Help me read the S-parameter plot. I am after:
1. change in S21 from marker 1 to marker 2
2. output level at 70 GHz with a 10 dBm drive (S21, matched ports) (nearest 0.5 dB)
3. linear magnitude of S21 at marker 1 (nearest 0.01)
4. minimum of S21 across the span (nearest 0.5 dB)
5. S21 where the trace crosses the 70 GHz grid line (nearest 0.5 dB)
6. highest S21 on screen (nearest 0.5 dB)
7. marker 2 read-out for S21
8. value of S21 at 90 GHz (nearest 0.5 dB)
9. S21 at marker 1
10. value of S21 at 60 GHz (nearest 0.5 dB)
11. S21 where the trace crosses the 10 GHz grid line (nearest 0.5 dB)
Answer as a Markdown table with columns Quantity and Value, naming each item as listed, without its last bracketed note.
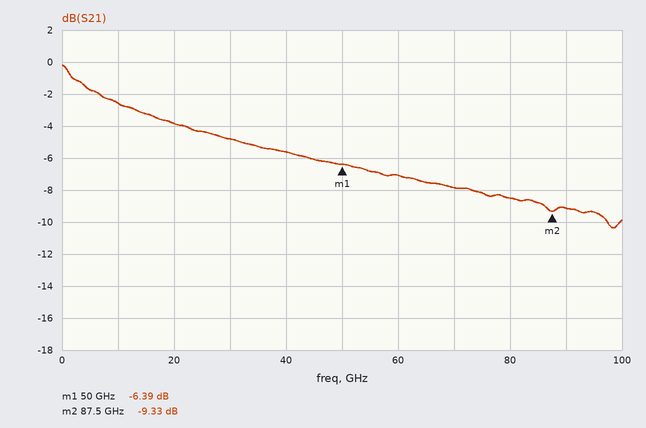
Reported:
| Quantity | Value |
|---|---|
| change in S21 from marker 1 to marker 2 | -2.94 dB |
| output level at 70 GHz with a 10 dBm drive (S21, matched ports) | 2.0 dBm |
| linear magnitude of S21 at marker 1 | 0.48 |
| minimum of S21 across the span | -10.5 dB |
| S21 where the trace crosses the 70 GHz grid line | -8.0 dB |
| highest S21 on screen | 0.0 dB |
| marker 2 read-out for S21 | -9.33 dB |
| value of S21 at 90 GHz | -9.0 dB |
| S21 at marker 1 | -6.39 dB |
| value of S21 at 60 GHz | -7.0 dB |
| S21 where the trace crosses the 10 GHz grid line | -2.5 dB |
